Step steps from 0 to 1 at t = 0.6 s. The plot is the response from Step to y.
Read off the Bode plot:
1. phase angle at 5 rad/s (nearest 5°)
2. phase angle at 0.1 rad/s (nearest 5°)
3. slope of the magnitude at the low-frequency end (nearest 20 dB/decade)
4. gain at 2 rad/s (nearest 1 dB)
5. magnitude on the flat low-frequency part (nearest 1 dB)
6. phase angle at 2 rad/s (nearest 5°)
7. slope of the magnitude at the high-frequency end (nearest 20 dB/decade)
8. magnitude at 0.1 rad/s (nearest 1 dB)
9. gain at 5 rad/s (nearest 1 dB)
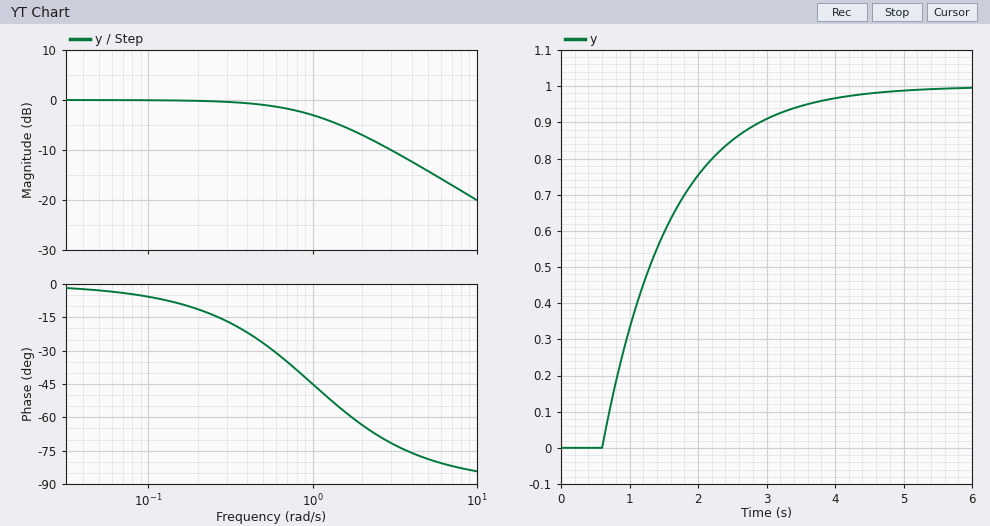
-80°
-5°
0 dB/decade
-7 dB
0 dB
-65°
-20 dB/decade
0 dB
-14 dB
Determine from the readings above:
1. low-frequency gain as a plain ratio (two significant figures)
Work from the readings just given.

1.0
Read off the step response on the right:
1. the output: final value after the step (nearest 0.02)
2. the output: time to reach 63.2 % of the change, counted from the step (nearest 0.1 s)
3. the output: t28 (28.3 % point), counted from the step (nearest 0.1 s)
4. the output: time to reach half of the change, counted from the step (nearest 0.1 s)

1.00
1.0 s
0.3 s
0.7 s
